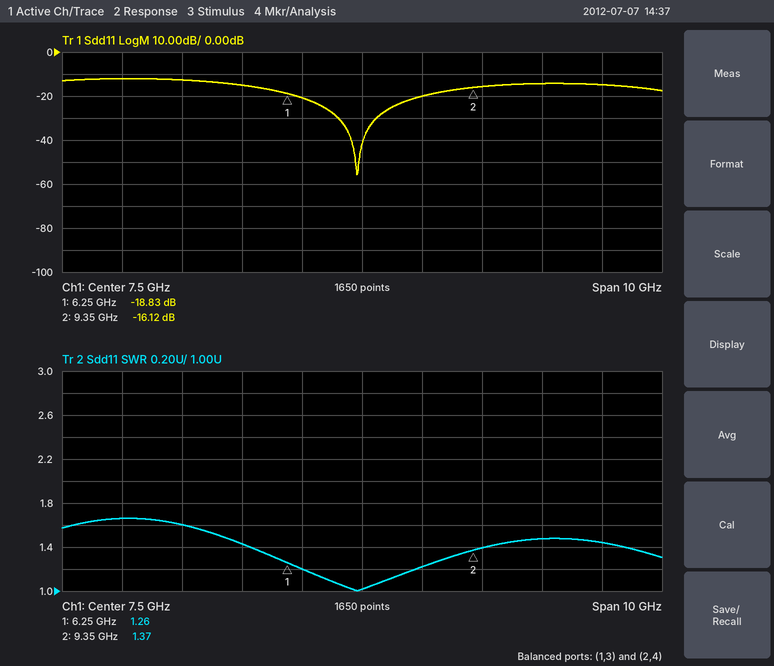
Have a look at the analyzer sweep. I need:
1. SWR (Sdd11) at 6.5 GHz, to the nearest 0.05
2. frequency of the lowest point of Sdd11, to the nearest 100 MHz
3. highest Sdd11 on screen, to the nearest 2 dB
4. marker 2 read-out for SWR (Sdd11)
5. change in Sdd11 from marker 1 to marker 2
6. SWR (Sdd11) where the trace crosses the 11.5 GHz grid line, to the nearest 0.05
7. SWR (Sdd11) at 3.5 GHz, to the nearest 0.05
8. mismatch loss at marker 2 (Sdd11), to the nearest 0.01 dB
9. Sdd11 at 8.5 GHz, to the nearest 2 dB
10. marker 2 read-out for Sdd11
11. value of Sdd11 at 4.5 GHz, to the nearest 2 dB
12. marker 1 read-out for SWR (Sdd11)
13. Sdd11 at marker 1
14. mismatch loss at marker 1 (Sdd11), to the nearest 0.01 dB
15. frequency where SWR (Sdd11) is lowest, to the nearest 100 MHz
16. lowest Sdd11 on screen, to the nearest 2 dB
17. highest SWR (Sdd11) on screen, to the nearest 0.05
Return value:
1.20
7.4 GHz
-12 dB
1.37
2.71 dB
1.45
1.65
0.11 dB
-20 dB
-16.12 dB
-12 dB
1.26
-18.83 dB
0.06 dB
7.4 GHz
-56 dB
1.65
